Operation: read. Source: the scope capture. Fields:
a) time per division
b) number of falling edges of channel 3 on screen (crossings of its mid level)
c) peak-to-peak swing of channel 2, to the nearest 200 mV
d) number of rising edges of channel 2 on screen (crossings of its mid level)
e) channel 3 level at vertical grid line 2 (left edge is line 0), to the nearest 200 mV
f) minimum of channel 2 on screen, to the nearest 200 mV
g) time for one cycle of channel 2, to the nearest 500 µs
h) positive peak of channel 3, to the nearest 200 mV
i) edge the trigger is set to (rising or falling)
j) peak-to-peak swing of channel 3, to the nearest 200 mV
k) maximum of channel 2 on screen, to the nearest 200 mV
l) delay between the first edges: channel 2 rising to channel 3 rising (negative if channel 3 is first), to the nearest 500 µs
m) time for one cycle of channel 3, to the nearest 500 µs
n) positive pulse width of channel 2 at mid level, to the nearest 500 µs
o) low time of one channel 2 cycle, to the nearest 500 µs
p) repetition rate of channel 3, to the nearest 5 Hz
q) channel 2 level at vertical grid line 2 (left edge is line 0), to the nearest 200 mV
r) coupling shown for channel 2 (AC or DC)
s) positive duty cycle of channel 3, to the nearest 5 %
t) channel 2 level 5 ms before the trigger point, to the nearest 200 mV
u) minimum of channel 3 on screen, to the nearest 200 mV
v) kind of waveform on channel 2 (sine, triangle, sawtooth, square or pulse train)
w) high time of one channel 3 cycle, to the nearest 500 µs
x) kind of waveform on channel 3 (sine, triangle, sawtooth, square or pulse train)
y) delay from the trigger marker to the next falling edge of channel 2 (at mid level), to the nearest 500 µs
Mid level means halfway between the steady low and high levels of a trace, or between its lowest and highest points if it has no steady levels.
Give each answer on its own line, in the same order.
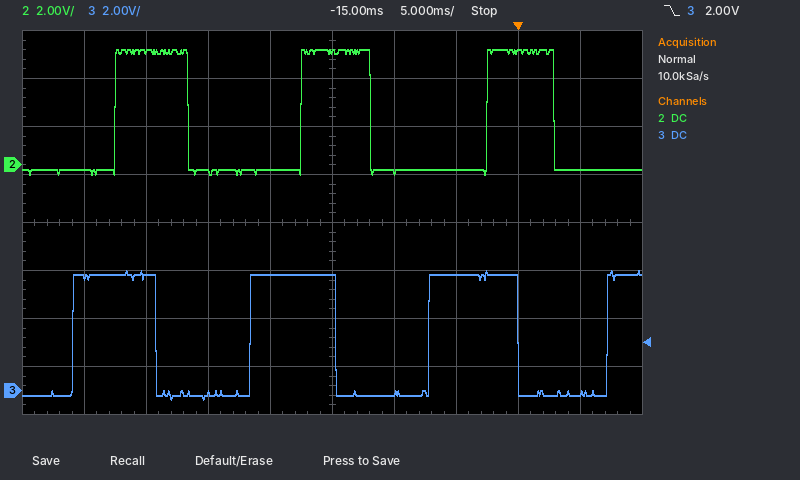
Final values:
5 ms
3
5.2 V
3
4.8 V
-400 mV
15.0 ms
5.0 V
falling
5.4 V
4.8 V
-3.5 ms
14.5 ms
5.5 ms
9.5 ms
70 Hz
4.8 V
DC
50 %
-200 mV
-400 mV
pulse train
7.0 ms
square
3.0 ms
